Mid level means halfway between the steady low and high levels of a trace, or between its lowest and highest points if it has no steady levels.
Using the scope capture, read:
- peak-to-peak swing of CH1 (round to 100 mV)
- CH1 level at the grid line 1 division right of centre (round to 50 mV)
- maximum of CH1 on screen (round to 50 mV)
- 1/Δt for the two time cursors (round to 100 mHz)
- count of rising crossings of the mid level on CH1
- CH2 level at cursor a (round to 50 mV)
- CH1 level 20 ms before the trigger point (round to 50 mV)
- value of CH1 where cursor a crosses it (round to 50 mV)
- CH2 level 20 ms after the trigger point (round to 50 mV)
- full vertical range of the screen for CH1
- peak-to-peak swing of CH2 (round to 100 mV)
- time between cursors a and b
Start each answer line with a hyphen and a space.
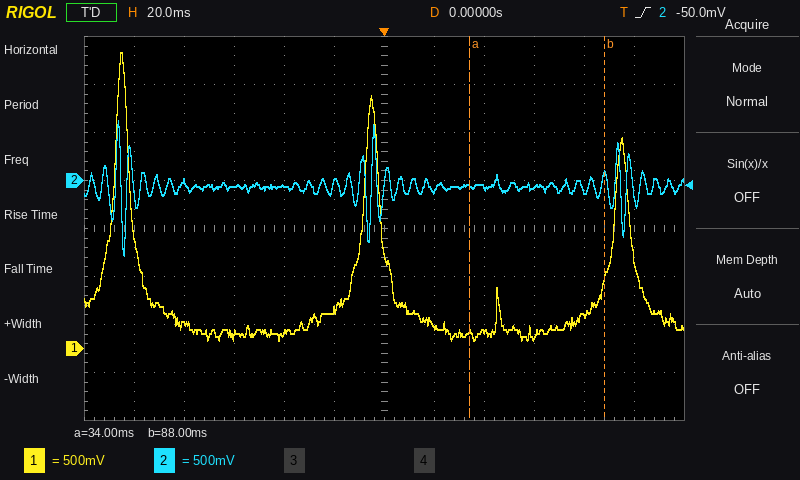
- 3.00 V
- 250 mV
- 3.10 V
- 18.5 Hz
- 3
- -50 mV
- 400 mV
- 150 mV
- -100 mV
- 4 V
- 1.40 V
- 54 ms
